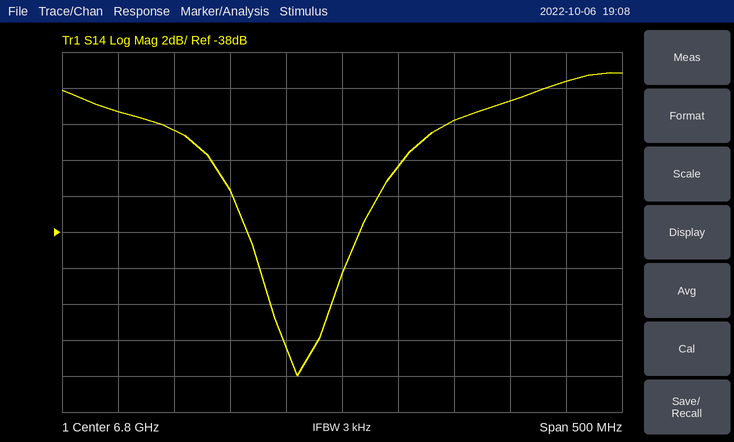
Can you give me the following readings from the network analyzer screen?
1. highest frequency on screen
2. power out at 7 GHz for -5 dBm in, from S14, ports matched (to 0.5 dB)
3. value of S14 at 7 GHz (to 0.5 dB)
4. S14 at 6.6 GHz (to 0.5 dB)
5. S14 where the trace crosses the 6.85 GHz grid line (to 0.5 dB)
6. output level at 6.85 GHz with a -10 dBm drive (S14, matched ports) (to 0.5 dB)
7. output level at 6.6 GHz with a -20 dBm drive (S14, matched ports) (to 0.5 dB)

7.05 GHz
-34.5 dBm
-29.5 dB
-31.5 dB
-34.5 dB
-44.5 dBm
-51.5 dBm
